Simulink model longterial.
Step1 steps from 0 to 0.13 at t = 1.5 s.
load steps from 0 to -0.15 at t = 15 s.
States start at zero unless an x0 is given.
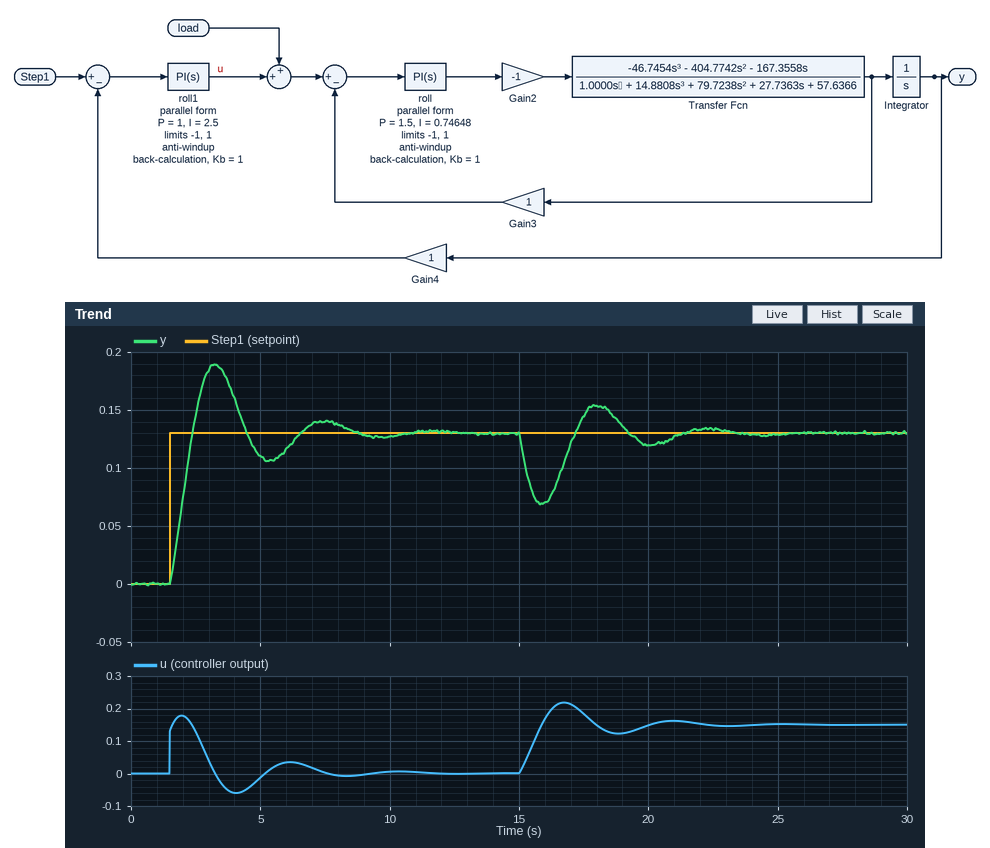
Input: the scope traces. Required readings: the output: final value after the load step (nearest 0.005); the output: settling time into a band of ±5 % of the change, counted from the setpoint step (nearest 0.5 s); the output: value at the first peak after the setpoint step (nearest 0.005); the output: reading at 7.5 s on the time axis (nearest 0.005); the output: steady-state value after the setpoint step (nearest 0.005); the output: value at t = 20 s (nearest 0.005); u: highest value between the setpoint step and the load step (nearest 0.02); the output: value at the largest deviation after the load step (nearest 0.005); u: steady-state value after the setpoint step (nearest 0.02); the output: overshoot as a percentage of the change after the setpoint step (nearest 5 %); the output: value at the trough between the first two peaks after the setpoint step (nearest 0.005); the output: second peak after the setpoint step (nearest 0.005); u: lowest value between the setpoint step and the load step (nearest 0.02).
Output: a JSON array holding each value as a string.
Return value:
["0.130", "6.5 s", "0.190", "0.140", "0.130", "0.120", "0.18", "0.070", "0.00", "45 %", "0.105", "0.140", "-0.06"]
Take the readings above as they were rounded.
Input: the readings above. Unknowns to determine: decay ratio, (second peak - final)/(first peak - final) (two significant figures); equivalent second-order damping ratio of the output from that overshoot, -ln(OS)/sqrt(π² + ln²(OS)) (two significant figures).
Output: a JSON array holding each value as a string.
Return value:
["0.17", "0.25"]
